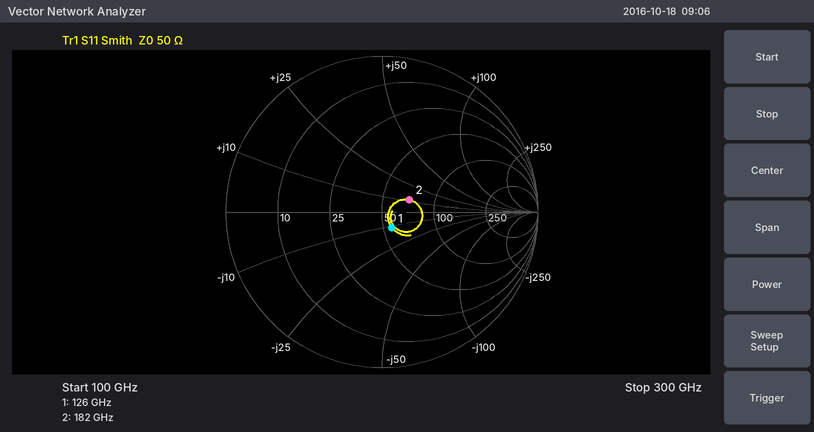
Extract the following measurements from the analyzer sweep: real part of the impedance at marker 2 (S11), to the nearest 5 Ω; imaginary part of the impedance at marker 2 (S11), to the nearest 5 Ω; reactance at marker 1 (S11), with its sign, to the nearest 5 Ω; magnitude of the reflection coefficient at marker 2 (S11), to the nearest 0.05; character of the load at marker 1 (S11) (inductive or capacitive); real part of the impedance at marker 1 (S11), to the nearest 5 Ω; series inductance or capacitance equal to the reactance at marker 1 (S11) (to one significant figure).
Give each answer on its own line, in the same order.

70 Ω
+10 Ω
-10 Ω
0.20
capacitive
55 Ω
100 fF
